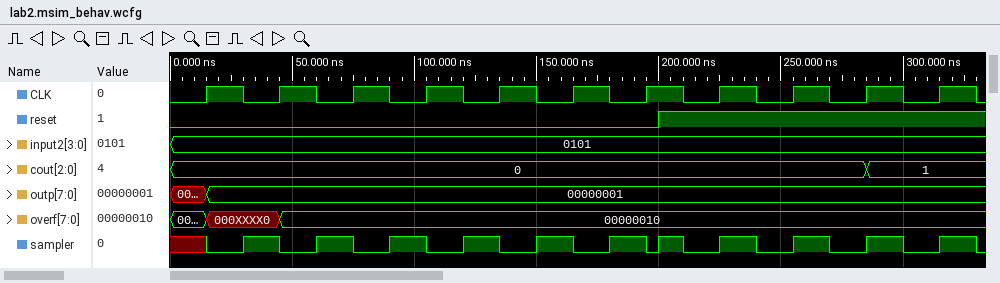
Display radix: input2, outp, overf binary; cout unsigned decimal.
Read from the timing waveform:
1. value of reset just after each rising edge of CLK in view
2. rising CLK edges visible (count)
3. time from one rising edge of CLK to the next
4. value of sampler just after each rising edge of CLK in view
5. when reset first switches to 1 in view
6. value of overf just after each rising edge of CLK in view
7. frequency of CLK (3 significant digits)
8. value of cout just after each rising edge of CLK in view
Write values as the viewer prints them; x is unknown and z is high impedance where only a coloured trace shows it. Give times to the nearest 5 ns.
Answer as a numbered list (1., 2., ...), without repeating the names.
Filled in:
1. 0 0 0 0 0 0 0 1 1 1 1
2. 11
3. 30 ns
4. 0 0 0 0 0 0 0 1 1 1 1
5. 200 ns
6. 000XXXX0, 00000010, 00000010, 00000010, 00000010, 00000010, 00000010, 00000010, 00000010, 00000010, 00000010
7. 33.3 MHz
8. 0, 0, 0, 0, 0, 0, 0, 0, 0, 1, 1
